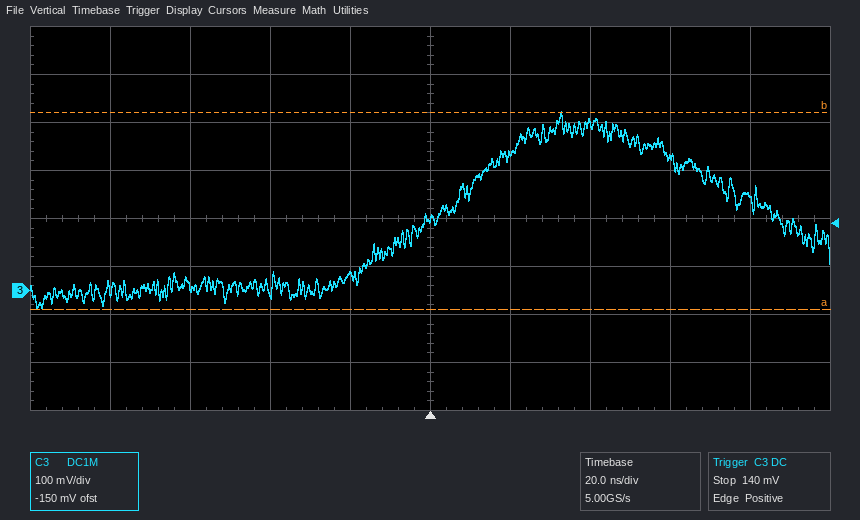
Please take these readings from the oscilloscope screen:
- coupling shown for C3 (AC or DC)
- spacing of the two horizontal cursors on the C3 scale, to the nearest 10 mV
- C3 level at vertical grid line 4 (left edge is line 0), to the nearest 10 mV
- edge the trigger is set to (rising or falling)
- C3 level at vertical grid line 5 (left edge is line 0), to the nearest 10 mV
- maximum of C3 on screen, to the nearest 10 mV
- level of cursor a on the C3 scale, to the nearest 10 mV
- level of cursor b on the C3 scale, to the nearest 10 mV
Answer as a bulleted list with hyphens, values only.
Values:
- DC
- 410 mV
- 30 mV
- rising
- 150 mV
- 370 mV
- -40 mV
- 370 mV
